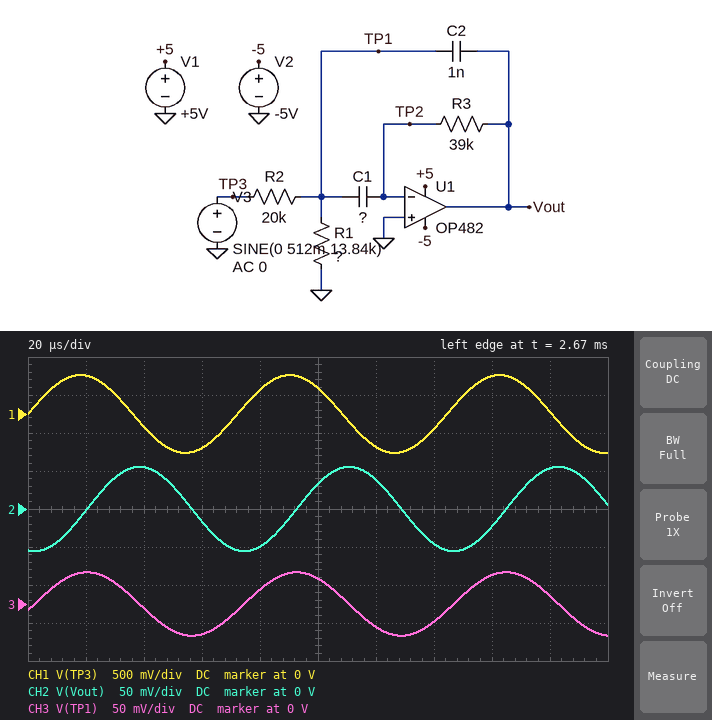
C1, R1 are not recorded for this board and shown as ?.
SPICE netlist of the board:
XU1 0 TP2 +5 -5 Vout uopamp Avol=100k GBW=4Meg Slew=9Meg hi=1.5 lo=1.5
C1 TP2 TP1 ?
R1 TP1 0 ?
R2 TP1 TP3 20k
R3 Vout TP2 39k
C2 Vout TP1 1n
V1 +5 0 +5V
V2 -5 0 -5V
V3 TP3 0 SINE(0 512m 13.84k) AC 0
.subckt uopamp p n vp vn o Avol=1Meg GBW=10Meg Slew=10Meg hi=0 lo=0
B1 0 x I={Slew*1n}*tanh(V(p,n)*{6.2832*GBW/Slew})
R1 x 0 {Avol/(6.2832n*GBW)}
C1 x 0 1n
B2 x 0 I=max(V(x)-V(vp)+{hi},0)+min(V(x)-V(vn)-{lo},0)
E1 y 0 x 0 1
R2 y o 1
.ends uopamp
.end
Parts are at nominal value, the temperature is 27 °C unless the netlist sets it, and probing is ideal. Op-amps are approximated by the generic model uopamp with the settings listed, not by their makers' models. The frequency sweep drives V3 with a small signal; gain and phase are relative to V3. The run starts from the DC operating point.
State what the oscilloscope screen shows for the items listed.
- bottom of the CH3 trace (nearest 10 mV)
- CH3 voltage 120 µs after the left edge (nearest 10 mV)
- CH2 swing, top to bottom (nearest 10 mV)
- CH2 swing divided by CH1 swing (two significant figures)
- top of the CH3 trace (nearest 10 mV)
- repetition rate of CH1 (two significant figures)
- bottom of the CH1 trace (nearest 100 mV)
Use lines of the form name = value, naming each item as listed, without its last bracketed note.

bottom of the CH3 trace = -40 mV
CH3 voltage 120 µs after the left edge = -30 mV
CH2 swing, top to bottom = 110 mV
CH2 swing divided by CH1 swing = 0.11
top of the CH3 trace = 40 mV
repetition rate of CH1 = 14 kHz
bottom of the CH1 trace = -500 mV
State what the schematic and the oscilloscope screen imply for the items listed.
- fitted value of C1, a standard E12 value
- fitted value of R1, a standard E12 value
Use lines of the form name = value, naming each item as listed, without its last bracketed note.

fitted value of C1, a standard E12 value = 390 pF
fitted value of R1, a standard E12 value = 1.5 kΩ
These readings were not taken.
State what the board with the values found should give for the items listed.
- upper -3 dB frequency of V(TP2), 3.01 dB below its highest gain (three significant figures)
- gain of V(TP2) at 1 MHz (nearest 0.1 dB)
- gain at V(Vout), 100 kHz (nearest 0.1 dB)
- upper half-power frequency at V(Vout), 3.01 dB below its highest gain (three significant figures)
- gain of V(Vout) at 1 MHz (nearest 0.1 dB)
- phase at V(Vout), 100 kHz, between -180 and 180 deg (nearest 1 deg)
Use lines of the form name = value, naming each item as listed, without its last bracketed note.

upper -3 dB frequency of V(TP2), 3.01 dB below its highest gain = 47.8 kHz
gain of V(TP2) at 1 MHz = -54.5 dB
gain at V(Vout), 100 kHz = -21.3 dB
upper half-power frequency at V(Vout), 3.01 dB below its highest gain = 41.9 kHz
gain of V(Vout) at 1 MHz = -42.5 dB
phase at V(Vout), 100 kHz, between -180 and 180 deg = 98 deg
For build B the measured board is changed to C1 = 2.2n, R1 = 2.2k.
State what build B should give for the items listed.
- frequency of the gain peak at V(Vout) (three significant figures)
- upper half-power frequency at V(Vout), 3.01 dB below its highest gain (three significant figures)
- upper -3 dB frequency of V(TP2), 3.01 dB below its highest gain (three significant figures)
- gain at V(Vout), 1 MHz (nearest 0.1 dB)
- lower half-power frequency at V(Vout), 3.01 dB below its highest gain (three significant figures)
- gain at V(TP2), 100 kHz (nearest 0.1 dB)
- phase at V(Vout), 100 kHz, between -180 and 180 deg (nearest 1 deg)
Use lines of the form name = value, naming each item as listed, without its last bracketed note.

frequency of the gain peak at V(Vout) = 12.1 kHz
upper half-power frequency at V(Vout), 3.01 dB below its highest gain = 15.3 kHz
upper -3 dB frequency of V(TP2), 3.01 dB below its highest gain = 18.7 kHz
gain at V(Vout), 1 MHz = -42.4 dB
lower half-power frequency at V(Vout), 3.01 dB below its highest gain = 9.52 kHz
gain at V(TP2), 100 kHz = -54.1 dB
phase at V(Vout), 100 kHz, between -180 and 180 deg = 92 deg
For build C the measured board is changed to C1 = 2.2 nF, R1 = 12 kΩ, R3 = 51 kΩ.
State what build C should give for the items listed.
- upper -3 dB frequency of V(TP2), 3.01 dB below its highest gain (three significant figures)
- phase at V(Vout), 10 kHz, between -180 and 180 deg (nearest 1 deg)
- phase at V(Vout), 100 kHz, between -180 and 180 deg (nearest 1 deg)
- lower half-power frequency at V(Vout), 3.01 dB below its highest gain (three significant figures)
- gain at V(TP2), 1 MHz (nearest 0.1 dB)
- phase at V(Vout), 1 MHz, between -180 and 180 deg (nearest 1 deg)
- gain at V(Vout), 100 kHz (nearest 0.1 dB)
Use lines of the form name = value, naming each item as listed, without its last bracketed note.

upper -3 dB frequency of V(TP2), 3.01 dB below its highest gain = 1.45 MHz
phase at V(Vout), 10 kHz, between -180 and 180 deg = 123 deg
phase at V(Vout), 100 kHz, between -180 and 180 deg = 91 deg
lower half-power frequency at V(Vout), 3.01 dB below its highest gain = 3.66 kHz
gain at V(TP2), 1 MHz = -54.3 dB
phase at V(Vout), 1 MHz, between -180 and 180 deg = 76 deg
gain at V(Vout), 100 kHz = -22.0 dB
